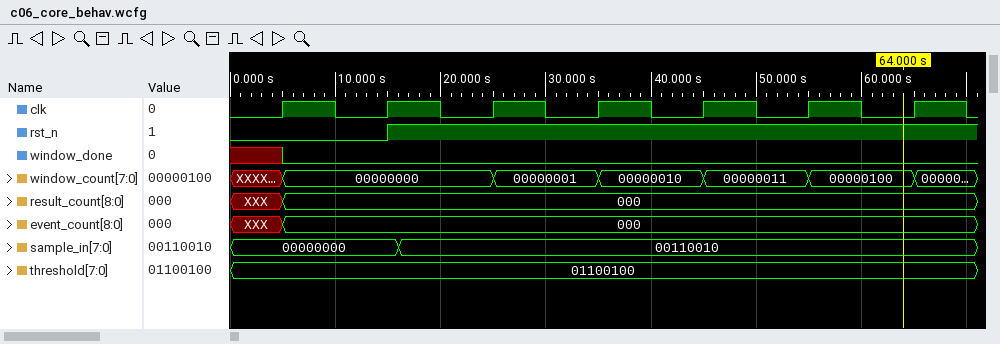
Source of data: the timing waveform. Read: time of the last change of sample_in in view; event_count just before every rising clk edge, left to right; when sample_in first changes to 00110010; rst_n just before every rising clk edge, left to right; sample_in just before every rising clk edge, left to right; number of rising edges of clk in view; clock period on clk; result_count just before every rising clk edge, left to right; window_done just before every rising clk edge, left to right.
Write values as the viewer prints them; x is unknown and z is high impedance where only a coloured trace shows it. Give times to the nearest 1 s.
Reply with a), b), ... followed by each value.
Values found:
a) 16 s
b) XXX, 000, 000, 000, 000, 000, 000
c) 16 s
d) 0 0 1 1 1 1 1
e) 00000000, 00000000, 00110010, 00110010, 00110010, 00110010, 00110010
f) 7
g) 10 s
h) XXX, 000, 000, 000, 000, 000, 000
i) x 0 0 0 0 0 0
